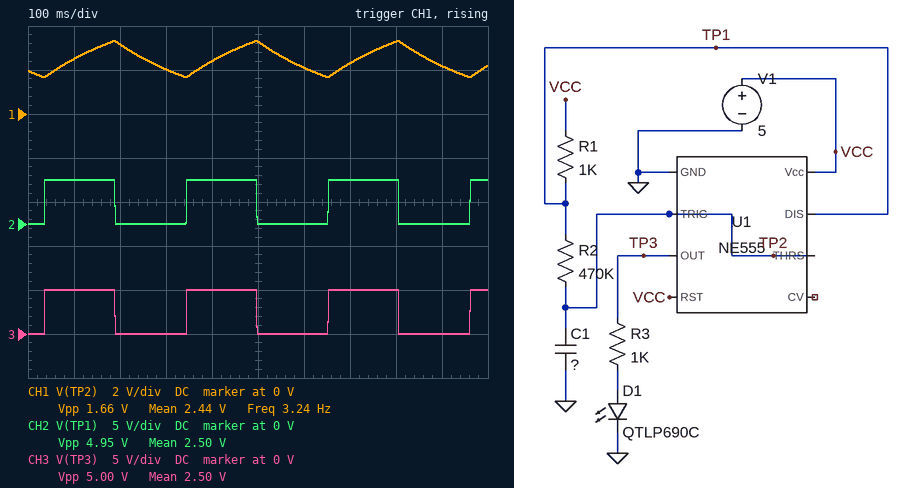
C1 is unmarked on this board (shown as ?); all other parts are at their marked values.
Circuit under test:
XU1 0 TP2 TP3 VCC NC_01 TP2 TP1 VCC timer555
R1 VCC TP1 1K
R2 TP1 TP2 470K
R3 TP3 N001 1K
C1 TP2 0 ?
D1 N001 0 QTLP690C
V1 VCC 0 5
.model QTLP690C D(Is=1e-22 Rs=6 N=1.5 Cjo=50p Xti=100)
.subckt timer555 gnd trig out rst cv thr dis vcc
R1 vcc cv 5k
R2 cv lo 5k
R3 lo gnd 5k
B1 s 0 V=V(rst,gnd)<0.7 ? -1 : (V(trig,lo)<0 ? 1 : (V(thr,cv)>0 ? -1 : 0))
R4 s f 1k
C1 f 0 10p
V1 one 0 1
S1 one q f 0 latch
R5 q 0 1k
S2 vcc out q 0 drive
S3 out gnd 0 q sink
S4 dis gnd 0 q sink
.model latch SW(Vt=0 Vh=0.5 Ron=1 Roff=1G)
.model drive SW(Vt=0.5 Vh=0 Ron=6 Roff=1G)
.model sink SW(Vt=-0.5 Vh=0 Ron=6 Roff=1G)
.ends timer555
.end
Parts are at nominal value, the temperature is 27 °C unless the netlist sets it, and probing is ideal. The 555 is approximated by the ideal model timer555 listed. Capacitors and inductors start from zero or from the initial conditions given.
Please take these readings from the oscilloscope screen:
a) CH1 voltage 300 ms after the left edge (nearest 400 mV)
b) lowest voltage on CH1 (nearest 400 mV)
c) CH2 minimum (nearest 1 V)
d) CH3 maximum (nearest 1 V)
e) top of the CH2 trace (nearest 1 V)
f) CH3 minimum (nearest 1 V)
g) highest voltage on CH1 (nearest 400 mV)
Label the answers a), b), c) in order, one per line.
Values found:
a) 2.0 V
b) 1.6 V
c) 0 V
d) 5 V
e) 5 V
f) 0 V
g) 3.2 V
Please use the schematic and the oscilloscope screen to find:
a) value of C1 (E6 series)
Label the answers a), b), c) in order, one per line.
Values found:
a) 470 nF
